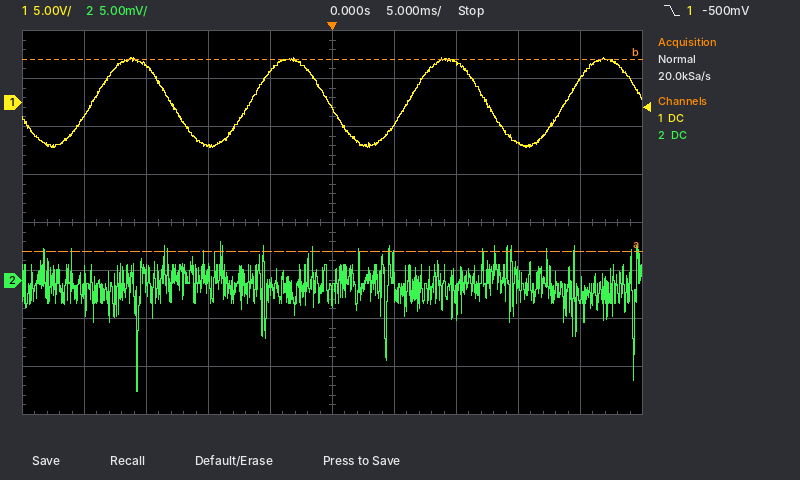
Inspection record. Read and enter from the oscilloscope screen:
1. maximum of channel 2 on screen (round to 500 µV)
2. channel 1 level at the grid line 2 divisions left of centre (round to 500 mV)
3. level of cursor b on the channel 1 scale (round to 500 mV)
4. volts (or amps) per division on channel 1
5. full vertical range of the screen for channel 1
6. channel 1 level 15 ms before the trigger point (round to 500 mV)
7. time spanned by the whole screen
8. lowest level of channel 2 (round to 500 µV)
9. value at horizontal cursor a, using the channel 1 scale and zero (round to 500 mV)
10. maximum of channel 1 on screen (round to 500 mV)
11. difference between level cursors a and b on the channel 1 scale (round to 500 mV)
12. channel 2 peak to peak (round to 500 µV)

4.0 mV
-4.5 V
4.5 V
5 V
40 V
4.0 V
50 ms
-11.5 mV
-15.5 V
4.5 V
20.0 V
15.5 mV
